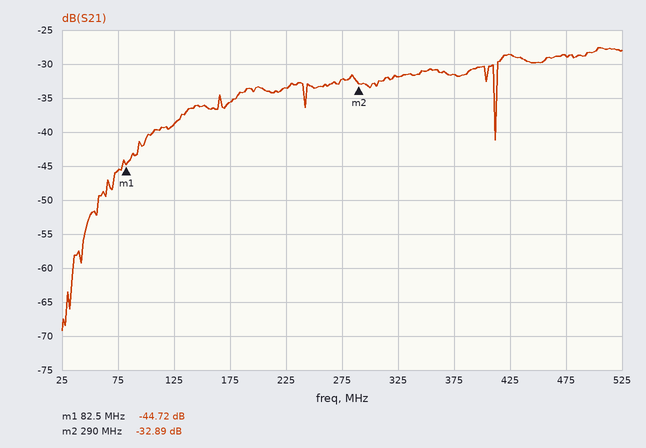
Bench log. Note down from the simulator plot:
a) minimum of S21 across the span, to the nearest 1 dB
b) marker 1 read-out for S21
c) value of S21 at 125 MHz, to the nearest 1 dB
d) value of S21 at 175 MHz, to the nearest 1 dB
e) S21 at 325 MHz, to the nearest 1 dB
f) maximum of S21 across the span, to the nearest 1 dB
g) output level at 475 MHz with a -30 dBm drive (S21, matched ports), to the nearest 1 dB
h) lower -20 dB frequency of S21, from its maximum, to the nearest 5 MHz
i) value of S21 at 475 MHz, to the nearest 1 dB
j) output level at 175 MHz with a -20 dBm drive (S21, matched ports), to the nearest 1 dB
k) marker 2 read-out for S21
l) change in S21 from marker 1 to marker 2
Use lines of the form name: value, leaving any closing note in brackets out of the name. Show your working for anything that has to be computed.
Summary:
minimum of S21 across the span, to the nearest 1 dB: -69 dB
marker 1 read-out for S21: -44.72 dB
value of S21 at 125 MHz, to the nearest 1 dB: -39 dB
value of S21 at 175 MHz, to the nearest 1 dB: -36 dB
S21 at 325 MHz, to the nearest 1 dB: -32 dB
maximum of S21 across the span, to the nearest 1 dB: -28 dB
output level at 475 MHz with a -30 dBm drive (S21, matched ports), to the nearest 1 dB: -30 dBm + (-29 dB) = -59 dBm
lower -20 dB frequency of S21, from its maximum, to the nearest 5 MHz: 70 MHz
value of S21 at 475 MHz, to the nearest 1 dB: -29 dB
output level at 175 MHz with a -20 dBm drive (S21, matched ports), to the nearest 1 dB: -20 dBm + (-36 dB) = -56 dBm
marker 2 read-out for S21: -32.89 dB
change in S21 from marker 1 to marker 2: -32.89 − (-44.72) = 11.83 dB
